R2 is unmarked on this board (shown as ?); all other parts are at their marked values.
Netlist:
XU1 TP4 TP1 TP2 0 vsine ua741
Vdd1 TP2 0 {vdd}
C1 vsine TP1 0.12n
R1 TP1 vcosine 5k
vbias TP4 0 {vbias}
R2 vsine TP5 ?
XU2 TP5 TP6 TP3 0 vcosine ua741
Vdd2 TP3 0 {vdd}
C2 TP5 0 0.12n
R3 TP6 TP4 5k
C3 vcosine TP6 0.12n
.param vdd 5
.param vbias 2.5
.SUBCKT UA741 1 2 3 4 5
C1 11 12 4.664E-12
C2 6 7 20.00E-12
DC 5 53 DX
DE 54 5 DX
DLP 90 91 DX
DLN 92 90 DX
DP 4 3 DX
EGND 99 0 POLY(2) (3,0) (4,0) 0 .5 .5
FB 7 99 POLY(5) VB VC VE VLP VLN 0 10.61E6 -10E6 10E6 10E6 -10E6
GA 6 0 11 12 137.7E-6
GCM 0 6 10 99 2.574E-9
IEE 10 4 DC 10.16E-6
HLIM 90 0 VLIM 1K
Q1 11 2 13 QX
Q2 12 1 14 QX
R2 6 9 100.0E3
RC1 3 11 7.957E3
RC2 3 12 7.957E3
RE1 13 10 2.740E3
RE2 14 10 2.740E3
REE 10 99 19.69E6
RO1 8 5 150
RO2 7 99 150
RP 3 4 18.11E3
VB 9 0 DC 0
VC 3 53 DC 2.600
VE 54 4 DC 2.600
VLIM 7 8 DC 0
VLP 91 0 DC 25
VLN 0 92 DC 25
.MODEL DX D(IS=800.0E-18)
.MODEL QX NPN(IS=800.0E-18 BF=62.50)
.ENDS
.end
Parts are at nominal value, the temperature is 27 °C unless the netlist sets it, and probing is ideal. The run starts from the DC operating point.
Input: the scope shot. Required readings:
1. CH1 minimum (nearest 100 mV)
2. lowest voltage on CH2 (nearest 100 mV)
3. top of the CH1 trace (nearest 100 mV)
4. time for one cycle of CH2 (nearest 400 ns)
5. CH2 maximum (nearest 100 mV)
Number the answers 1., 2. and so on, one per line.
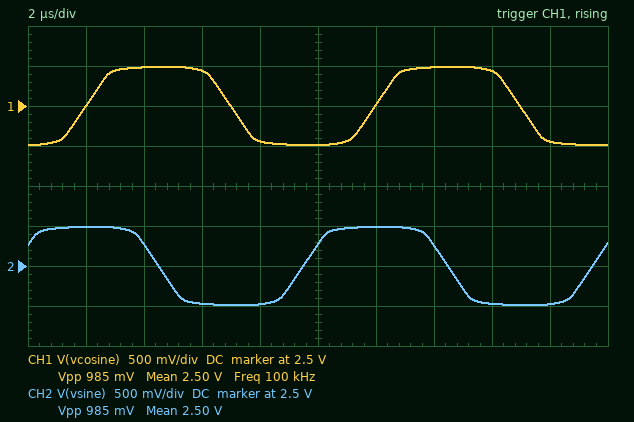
1. 2.0 V
2. 2.0 V
3. 3.0 V
4. 10.0 µs
5. 3.0 V
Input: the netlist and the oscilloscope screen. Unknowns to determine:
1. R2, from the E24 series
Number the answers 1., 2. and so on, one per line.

1. 4.7 kΩ
